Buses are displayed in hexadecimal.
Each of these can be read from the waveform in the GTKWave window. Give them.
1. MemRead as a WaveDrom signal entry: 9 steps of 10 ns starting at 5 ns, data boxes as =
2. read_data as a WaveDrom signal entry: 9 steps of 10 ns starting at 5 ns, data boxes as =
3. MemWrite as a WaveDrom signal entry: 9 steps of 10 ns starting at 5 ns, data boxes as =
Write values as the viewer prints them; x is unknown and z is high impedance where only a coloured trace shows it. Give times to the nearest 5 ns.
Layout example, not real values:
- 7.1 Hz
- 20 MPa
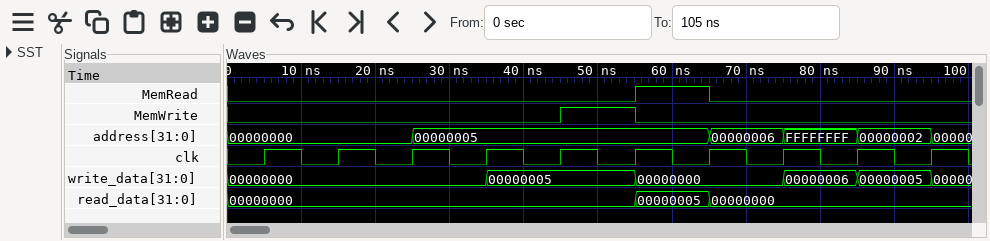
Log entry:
- {name: 'MemRead', wave: '0....10..'}
- {name: 'read_data', wave: '=....==..', data: '00000000 00000005 00000000'}
- {name: 'MemWrite', wave: '0...10...'}
